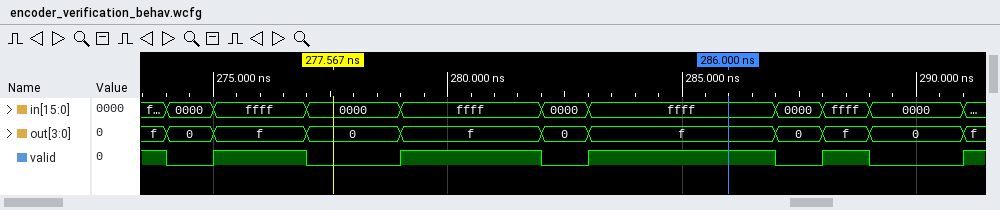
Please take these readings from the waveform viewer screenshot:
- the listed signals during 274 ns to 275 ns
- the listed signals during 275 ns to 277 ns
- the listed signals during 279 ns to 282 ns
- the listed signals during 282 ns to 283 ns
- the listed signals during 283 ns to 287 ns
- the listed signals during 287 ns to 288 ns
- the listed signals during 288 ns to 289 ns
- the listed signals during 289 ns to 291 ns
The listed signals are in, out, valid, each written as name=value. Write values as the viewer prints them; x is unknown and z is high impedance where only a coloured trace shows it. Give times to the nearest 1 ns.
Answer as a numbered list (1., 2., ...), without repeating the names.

1. in=0000, out=0, valid=0
2. in=ffff, out=f, valid=1
3. in=ffff, out=f, valid=1
4. in=0000, out=0, valid=0
5. in=ffff, out=f, valid=1
6. in=0000, out=0, valid=0
7. in=ffff, out=f, valid=1
8. in=0000, out=0, valid=0
